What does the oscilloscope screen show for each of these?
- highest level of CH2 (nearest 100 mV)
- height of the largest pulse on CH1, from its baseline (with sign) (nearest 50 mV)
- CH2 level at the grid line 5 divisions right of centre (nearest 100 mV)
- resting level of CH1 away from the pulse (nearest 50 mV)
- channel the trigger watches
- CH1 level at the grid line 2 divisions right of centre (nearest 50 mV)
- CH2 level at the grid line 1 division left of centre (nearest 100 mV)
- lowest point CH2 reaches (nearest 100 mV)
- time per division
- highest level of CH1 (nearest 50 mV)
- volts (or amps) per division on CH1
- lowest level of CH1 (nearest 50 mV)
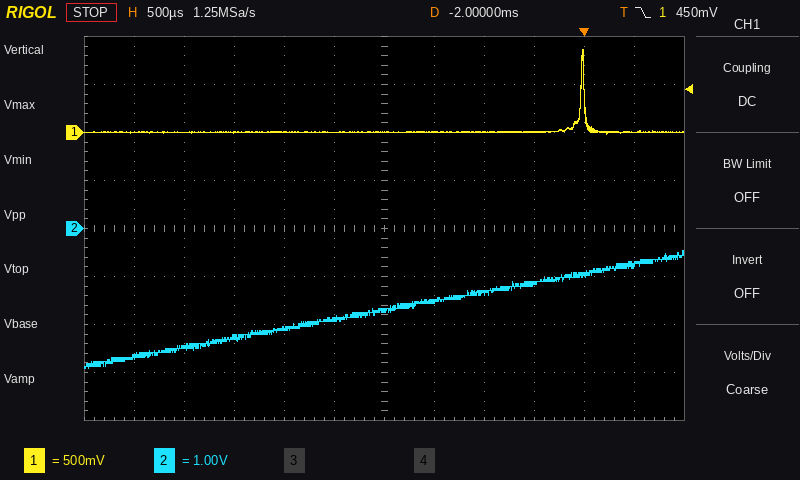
-500 mV
+850 mV
-800 mV
0 mV
CH1
0 mV
-1.9 V
-2.9 V
500 µs
850 mV
500 mV
0 mV
